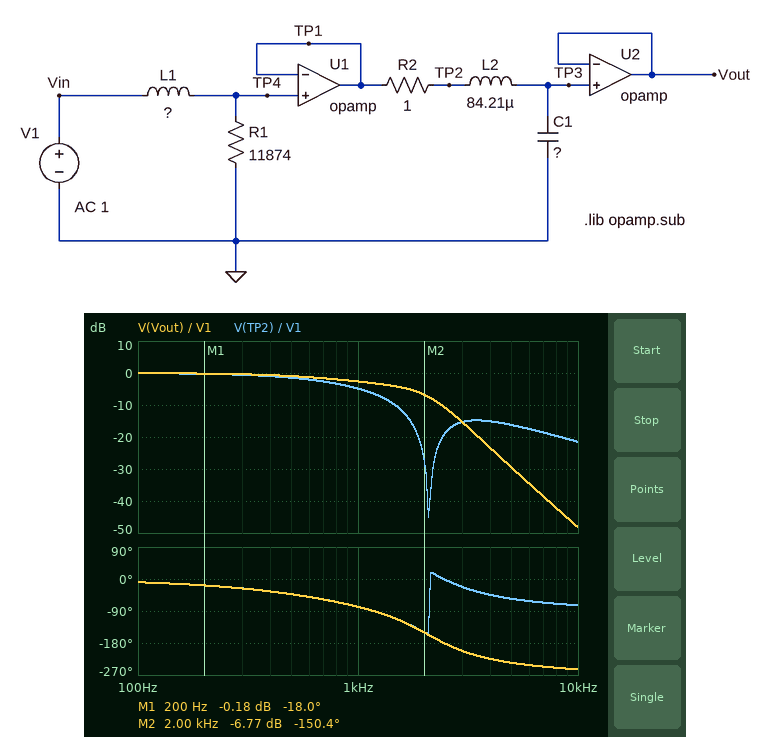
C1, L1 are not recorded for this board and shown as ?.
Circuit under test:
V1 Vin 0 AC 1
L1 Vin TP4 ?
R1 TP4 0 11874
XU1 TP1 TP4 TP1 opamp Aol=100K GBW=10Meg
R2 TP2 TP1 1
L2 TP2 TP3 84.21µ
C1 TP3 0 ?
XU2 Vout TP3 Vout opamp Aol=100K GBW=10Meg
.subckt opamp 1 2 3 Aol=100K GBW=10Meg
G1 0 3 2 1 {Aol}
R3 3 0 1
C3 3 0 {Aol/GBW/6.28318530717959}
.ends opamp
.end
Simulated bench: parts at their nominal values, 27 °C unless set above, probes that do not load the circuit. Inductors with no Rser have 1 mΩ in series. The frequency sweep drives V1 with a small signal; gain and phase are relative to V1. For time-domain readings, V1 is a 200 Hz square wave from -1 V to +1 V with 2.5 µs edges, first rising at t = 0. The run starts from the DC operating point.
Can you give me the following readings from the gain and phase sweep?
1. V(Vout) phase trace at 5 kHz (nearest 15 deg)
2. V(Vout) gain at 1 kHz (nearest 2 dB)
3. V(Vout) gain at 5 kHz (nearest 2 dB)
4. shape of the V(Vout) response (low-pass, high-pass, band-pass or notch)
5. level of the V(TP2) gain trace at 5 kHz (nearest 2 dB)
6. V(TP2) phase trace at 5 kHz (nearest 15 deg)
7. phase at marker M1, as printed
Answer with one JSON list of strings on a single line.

["-240 deg", "-2 dB", "-30 dB", "low-pass", "-16 dB", "-60 deg", "-18.0 deg"]
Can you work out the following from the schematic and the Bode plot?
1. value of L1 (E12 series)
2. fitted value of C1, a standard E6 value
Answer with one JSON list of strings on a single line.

["2.2 H", "68 µF"]
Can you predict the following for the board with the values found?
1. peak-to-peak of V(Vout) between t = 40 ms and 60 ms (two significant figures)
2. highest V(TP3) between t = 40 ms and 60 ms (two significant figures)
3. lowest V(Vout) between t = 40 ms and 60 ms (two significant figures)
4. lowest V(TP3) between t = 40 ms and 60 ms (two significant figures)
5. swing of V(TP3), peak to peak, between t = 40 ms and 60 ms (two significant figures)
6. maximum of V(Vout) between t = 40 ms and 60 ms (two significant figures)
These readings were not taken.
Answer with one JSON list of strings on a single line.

["2.0 V", "1.0 V", "-1.0 V", "-1.0 V", "2.0 V", "1.0 V"]
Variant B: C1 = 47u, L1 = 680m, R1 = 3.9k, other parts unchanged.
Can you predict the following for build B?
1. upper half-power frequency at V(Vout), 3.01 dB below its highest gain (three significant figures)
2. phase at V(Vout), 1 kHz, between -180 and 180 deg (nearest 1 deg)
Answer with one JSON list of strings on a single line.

["1.22 kHz", "-67 deg"]
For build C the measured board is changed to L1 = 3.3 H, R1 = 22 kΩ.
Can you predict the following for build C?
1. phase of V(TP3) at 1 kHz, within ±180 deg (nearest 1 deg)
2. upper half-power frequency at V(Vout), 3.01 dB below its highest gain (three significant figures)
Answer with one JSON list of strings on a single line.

["-72 deg", "1.53 kHz"]
